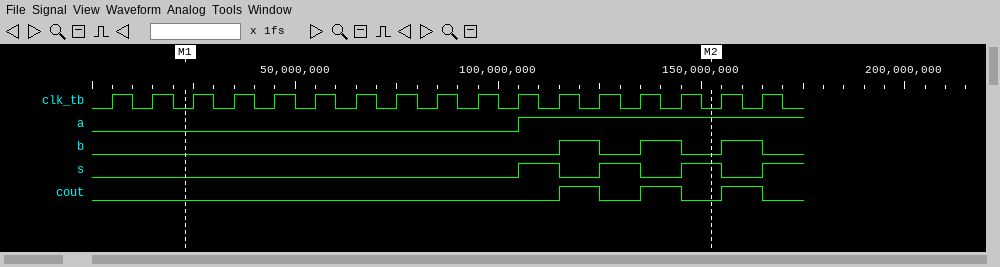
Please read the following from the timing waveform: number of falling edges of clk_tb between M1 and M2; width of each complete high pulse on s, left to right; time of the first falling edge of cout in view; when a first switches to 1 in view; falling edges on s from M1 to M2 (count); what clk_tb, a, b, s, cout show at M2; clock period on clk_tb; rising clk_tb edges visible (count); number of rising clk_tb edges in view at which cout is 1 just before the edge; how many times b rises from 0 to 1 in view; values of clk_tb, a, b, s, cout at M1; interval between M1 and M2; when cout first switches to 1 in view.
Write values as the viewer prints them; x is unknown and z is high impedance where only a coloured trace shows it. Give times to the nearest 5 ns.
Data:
13
10 ns, 10 ns, 10 ns
125 ns
105 ns
2
clk_tb=0, a=1, b=0, s=1, cout=0
10 ns
17
3
3
clk_tb=0, a=0, b=0, s=0, cout=0
130 ns
115 ns
